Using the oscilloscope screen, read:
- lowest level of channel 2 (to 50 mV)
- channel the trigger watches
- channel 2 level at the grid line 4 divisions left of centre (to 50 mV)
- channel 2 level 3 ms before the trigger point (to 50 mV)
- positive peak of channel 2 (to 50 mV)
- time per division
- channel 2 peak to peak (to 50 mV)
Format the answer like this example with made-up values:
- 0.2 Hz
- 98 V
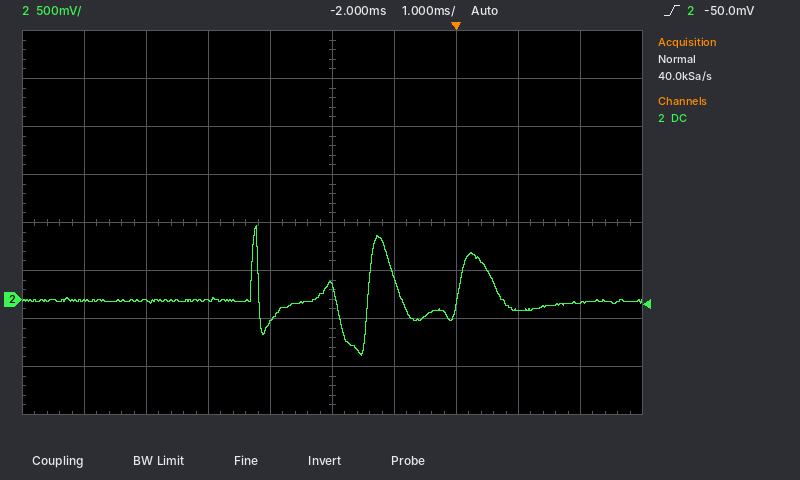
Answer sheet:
- -600 mV
- channel 2
- 0 mV
- -250 mV
- 750 mV
- 1 ms
- 1.35 V
